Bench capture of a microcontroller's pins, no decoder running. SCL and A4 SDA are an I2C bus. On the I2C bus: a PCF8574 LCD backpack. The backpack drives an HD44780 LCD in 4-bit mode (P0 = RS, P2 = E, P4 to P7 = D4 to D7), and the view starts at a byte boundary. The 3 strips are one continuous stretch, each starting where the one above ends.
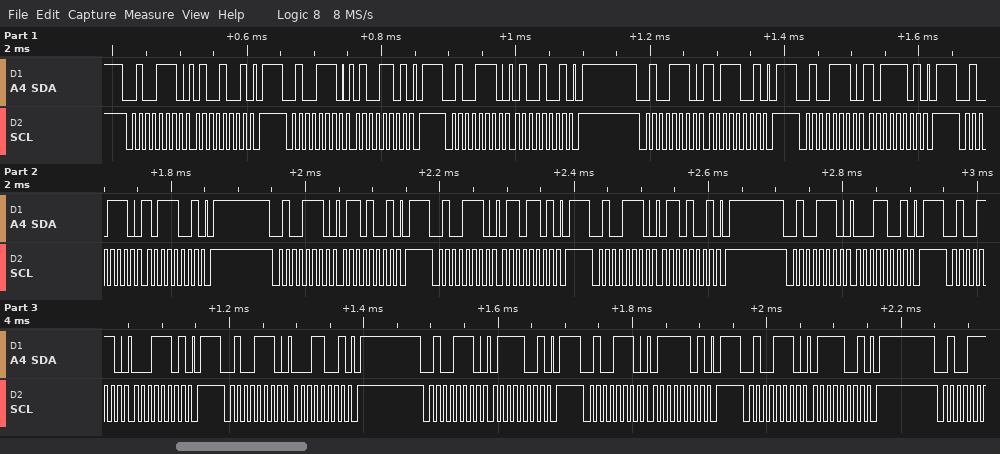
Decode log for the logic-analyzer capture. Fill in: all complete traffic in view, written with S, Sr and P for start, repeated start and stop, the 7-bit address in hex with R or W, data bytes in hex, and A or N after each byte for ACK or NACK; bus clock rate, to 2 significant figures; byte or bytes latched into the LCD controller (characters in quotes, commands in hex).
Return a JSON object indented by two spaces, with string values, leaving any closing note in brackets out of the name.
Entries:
{
  "all complete traffic in view, written with S, Sr and P for start, repeated start and stop, the 7-bit address in hex with R or W, data bytes in hex, and A or N after each byte for ACK or NACK": "S 27W A 49 A P S 27W A 4D A P S 27W A 49 A P S 27W A B9 A P S 27W A BD A P S 27W A B9 A P S 27W A 69 A P S 27W A 6D A P S 27W A 69 A P S 27W A 19 A P S 27W A 1D A P S 27W A 19 A P S 27W A 79 A P S 27W A 7D A P S 27W A 79 A P",
  "bus clock rate, to 2 significant figures": "100 kHz",
  "byte or bytes latched into the LCD controller": "'K' 'a'"
}
